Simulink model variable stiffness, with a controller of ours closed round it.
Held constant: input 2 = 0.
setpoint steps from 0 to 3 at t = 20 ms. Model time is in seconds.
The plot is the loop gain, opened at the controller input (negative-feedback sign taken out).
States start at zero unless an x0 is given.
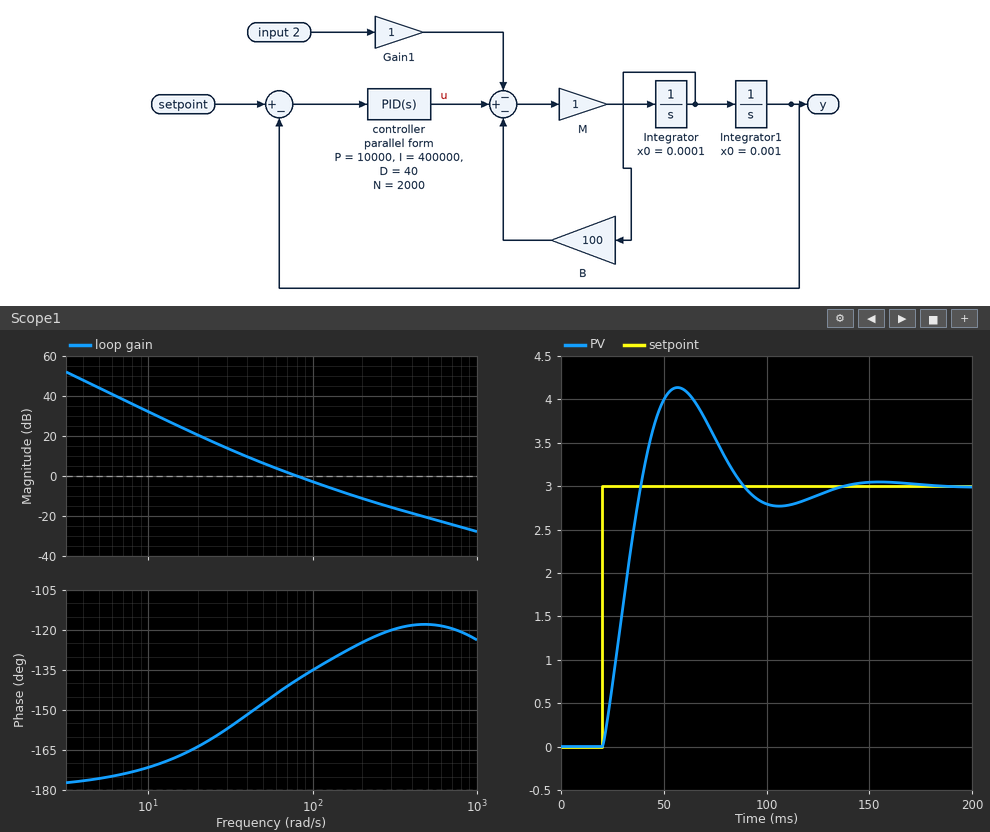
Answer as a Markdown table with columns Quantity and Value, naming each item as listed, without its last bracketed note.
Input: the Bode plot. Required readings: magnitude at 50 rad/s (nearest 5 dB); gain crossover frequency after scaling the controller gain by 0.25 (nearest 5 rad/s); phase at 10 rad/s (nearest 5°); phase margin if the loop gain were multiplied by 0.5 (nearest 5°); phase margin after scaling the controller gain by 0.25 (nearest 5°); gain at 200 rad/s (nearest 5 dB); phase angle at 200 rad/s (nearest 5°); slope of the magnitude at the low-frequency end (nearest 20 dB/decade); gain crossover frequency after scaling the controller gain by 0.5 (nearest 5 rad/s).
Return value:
| Quantity | Value |
|---|---|
| magnitude at 50 rad/s | 5 dB |
| gain crossover frequency after scaling the controller gain by 0.25 | 35 rad/s |
| phase at 10 rad/s | -170° |
| phase margin if the loop gain were multiplied by 0.5 | 35° |
| phase margin after scaling the controller gain by 0.25 | 25° |
| gain at 200 rad/s | -10 dB |
| phase angle at 200 rad/s | -125° |
| slope of the magnitude at the low-frequency end | -40 dB/decade |
| gain crossover frequency after scaling the controller gain by 0.5 | 50 rad/s |
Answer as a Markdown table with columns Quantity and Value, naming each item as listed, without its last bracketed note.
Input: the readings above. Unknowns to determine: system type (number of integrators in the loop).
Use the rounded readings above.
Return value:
| Quantity | Value |
|---|---|
| system type | 2 |
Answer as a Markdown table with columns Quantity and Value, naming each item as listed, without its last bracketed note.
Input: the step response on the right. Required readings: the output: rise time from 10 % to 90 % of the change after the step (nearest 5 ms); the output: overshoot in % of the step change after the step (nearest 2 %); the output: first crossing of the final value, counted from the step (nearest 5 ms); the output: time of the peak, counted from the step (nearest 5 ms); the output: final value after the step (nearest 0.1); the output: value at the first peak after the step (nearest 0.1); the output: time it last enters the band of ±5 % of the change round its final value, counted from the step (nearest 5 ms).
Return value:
| Quantity | Value |
|---|---|
| the output: rise time from 10 % to 90 % of the change after the step | 15 ms |
| the output: overshoot in % of the step change after the step | 38 % |
| the output: first crossing of the final value, counted from the step | 20 ms |
| the output: time of the peak, counted from the step | 35 ms |
| the output: final value after the step | 3.0 |
| the output: value at the first peak after the step | 4.1 |
| the output: time it last enters the band of ±5 % of the change round its final value, counted from the step | 100 ms |
